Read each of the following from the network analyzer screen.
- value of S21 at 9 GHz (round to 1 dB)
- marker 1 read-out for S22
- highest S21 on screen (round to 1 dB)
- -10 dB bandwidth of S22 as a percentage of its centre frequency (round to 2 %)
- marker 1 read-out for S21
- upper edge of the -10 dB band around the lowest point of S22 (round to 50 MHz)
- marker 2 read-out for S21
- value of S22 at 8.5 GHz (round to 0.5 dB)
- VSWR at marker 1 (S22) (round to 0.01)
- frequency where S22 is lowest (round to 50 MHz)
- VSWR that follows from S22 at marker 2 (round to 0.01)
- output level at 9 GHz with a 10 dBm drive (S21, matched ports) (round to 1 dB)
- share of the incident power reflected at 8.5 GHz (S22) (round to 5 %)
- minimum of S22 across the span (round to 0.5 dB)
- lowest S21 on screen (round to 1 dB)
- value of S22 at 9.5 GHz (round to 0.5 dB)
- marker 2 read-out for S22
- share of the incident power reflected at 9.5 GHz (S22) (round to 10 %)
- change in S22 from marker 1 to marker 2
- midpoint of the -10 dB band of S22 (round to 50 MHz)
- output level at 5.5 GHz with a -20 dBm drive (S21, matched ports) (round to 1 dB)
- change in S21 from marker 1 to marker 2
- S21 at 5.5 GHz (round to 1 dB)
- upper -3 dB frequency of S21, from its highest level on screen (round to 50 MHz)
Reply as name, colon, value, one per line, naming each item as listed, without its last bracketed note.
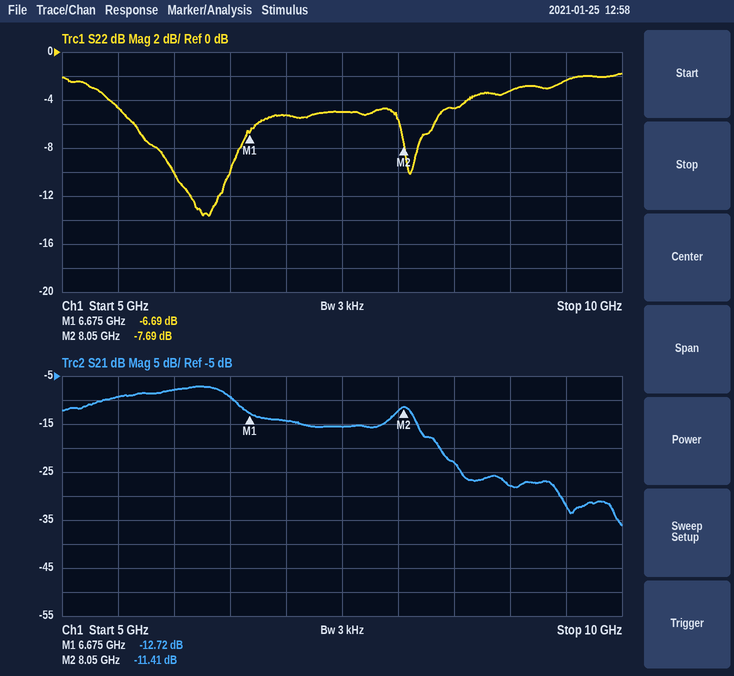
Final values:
value of S21 at 9 GHz: -28 dB
marker 1 read-out for S22: -6.69 dB
highest S21 on screen: -7 dB
-10 dB bandwidth of S22 as a percentage of its centre frequency: 8 %
marker 1 read-out for S21: -12.72 dB
upper edge of the -10 dB band around the lowest point of S22: 6.50 GHz
marker 2 read-out for S21: -11.41 dB
value of S22 at 8.5 GHz: -4.5 dB
VSWR at marker 1 (S22): 2.72
frequency where S22 is lowest: 6.25 GHz
VSWR that follows from S22 at marker 2: 2.40
output level at 9 GHz with a 10 dBm drive (S21, matched ports): -18 dBm
share of the incident power reflected at 8.5 GHz (S22): 35 %
minimum of S22 across the span: -13.5 dB
lowest S21 on screen: -36 dB
value of S22 at 9.5 GHz: -2.5 dB
marker 2 read-out for S22: -7.69 dB
share of the incident power reflected at 9.5 GHz (S22): 60 %
change in S22 from marker 1 to marker 2: -1.00 dB
midpoint of the -10 dB band of S22: 6.25 GHz
output level at 5.5 GHz with a -20 dBm drive (S21, matched ports): -29 dBm
change in S21 from marker 1 to marker 2: 1.31 dB
S21 at 5.5 GHz: -9 dB
upper -3 dB frequency of S21, from its highest level on screen: 6.55 GHz
